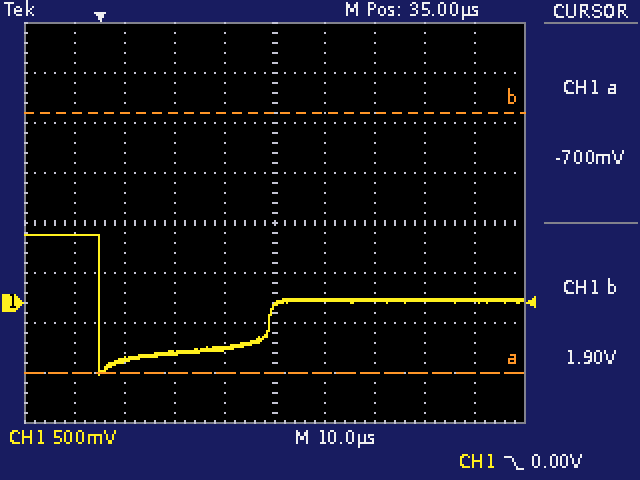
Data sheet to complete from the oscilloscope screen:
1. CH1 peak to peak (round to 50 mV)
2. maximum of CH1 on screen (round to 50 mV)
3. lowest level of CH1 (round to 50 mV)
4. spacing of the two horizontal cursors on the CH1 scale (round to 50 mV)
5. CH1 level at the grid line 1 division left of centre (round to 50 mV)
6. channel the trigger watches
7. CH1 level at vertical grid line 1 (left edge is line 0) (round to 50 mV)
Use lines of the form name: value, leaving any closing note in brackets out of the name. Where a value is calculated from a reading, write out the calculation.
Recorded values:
CH1 peak to peak: 700 mV − (-700 mV) = 1.40 V
maximum of CH1 on screen: 700 mV
lowest level of CH1: -700 mV
spacing of the two horizontal cursors on the CH1 scale: 2.60 V
CH1 level at the grid line 1 division left of centre: -450 mV
channel the trigger watches: CH1
CH1 level at vertical grid line 1 (left edge is line 0): 700 mV
